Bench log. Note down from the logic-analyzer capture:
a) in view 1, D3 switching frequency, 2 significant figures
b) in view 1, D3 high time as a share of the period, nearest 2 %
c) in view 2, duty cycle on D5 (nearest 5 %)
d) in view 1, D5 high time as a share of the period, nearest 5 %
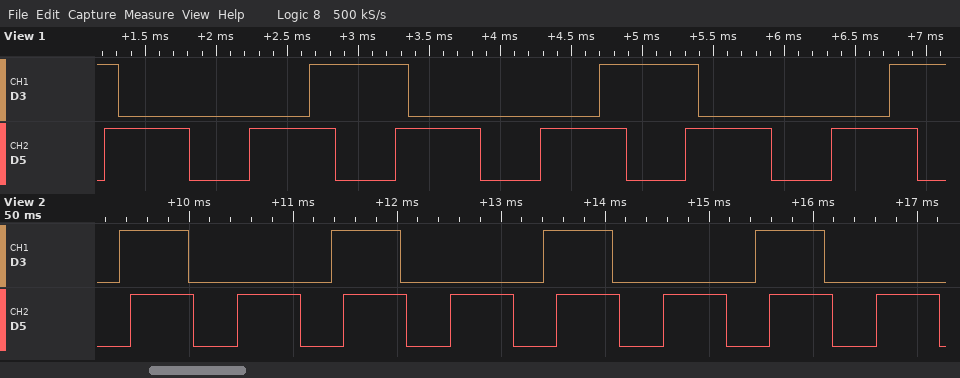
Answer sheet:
490 Hz
34 %
60 %
60 %
